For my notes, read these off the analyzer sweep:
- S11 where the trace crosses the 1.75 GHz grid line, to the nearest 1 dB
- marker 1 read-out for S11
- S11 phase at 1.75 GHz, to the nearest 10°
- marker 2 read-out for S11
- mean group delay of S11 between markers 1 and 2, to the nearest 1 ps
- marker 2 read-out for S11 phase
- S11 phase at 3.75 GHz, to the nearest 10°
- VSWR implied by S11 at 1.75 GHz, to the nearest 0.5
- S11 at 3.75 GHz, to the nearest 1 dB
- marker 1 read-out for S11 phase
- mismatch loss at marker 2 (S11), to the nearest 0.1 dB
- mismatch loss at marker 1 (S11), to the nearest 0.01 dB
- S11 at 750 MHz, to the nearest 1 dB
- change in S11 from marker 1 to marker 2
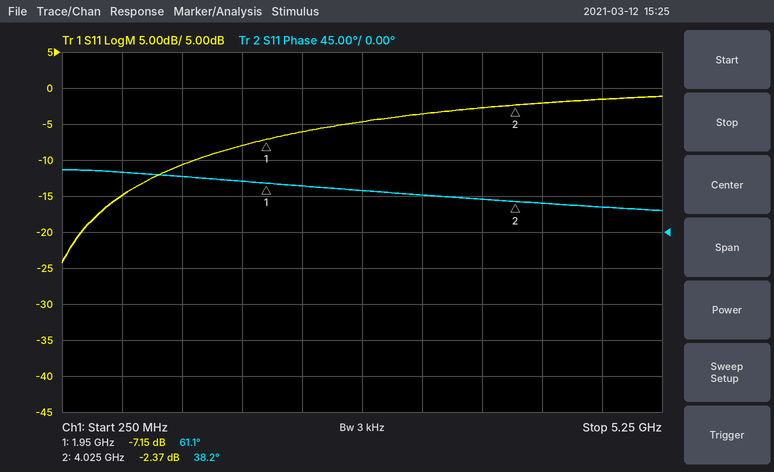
-8 dB
-7.15 dB
60°
-2.37 dB
31 ps
38.2°
40°
2.5
-3 dB
61.1°
3.8 dB
0.93 dB
-15 dB
4.78 dB
